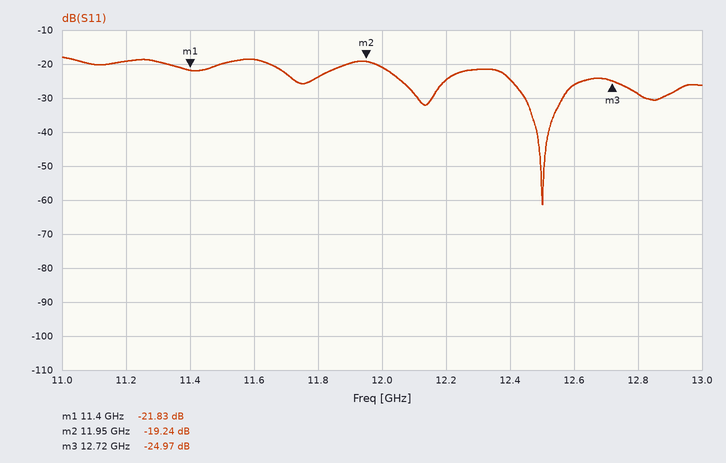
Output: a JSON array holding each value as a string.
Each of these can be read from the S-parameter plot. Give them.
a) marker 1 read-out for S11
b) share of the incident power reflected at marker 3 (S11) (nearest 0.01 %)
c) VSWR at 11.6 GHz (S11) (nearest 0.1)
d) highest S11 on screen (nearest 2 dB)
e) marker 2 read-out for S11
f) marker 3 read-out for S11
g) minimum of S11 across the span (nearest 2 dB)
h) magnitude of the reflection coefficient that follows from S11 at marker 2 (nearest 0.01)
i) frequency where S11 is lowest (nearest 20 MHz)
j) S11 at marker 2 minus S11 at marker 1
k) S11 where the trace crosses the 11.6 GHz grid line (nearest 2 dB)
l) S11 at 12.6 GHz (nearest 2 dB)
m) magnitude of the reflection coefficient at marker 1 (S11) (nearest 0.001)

["-21.83 dB", "0.32 %", "1.3", "-18 dB", "-19.24 dB", "-24.97 dB", "-62 dB", "0.11", "12.50 GHz", "2.59 dB", "-18 dB", "-26 dB", "0.081"]
